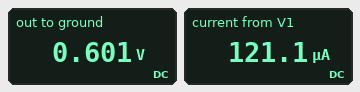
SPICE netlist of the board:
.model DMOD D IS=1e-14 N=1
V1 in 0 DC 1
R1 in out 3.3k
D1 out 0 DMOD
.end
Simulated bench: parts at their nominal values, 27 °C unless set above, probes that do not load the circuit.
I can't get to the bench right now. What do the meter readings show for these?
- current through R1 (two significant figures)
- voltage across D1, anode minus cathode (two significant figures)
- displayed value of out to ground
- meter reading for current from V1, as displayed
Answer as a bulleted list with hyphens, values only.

- 120 µA
- 600 mV
- 0.601 V
- 121.1 µA
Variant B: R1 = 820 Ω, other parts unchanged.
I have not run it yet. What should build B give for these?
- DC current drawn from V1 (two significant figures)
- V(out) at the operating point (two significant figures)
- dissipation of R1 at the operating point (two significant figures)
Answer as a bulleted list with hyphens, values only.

- 450 µA
- 630 mV
- 160 µW
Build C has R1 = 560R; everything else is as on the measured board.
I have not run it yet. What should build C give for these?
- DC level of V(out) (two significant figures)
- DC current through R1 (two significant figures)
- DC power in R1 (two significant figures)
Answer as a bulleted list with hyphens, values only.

- 640 mV
- 640 µA
- 230 µW
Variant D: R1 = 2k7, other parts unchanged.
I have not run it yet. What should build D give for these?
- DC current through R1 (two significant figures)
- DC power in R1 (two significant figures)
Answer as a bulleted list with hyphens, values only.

- 150 µA
- 58 µW
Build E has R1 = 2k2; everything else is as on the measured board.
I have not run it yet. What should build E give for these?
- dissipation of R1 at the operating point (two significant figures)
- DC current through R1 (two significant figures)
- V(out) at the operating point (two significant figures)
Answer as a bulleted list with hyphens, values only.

- 69 µW
- 180 µA
- 610 mV
